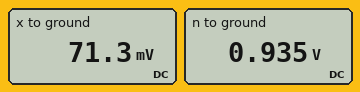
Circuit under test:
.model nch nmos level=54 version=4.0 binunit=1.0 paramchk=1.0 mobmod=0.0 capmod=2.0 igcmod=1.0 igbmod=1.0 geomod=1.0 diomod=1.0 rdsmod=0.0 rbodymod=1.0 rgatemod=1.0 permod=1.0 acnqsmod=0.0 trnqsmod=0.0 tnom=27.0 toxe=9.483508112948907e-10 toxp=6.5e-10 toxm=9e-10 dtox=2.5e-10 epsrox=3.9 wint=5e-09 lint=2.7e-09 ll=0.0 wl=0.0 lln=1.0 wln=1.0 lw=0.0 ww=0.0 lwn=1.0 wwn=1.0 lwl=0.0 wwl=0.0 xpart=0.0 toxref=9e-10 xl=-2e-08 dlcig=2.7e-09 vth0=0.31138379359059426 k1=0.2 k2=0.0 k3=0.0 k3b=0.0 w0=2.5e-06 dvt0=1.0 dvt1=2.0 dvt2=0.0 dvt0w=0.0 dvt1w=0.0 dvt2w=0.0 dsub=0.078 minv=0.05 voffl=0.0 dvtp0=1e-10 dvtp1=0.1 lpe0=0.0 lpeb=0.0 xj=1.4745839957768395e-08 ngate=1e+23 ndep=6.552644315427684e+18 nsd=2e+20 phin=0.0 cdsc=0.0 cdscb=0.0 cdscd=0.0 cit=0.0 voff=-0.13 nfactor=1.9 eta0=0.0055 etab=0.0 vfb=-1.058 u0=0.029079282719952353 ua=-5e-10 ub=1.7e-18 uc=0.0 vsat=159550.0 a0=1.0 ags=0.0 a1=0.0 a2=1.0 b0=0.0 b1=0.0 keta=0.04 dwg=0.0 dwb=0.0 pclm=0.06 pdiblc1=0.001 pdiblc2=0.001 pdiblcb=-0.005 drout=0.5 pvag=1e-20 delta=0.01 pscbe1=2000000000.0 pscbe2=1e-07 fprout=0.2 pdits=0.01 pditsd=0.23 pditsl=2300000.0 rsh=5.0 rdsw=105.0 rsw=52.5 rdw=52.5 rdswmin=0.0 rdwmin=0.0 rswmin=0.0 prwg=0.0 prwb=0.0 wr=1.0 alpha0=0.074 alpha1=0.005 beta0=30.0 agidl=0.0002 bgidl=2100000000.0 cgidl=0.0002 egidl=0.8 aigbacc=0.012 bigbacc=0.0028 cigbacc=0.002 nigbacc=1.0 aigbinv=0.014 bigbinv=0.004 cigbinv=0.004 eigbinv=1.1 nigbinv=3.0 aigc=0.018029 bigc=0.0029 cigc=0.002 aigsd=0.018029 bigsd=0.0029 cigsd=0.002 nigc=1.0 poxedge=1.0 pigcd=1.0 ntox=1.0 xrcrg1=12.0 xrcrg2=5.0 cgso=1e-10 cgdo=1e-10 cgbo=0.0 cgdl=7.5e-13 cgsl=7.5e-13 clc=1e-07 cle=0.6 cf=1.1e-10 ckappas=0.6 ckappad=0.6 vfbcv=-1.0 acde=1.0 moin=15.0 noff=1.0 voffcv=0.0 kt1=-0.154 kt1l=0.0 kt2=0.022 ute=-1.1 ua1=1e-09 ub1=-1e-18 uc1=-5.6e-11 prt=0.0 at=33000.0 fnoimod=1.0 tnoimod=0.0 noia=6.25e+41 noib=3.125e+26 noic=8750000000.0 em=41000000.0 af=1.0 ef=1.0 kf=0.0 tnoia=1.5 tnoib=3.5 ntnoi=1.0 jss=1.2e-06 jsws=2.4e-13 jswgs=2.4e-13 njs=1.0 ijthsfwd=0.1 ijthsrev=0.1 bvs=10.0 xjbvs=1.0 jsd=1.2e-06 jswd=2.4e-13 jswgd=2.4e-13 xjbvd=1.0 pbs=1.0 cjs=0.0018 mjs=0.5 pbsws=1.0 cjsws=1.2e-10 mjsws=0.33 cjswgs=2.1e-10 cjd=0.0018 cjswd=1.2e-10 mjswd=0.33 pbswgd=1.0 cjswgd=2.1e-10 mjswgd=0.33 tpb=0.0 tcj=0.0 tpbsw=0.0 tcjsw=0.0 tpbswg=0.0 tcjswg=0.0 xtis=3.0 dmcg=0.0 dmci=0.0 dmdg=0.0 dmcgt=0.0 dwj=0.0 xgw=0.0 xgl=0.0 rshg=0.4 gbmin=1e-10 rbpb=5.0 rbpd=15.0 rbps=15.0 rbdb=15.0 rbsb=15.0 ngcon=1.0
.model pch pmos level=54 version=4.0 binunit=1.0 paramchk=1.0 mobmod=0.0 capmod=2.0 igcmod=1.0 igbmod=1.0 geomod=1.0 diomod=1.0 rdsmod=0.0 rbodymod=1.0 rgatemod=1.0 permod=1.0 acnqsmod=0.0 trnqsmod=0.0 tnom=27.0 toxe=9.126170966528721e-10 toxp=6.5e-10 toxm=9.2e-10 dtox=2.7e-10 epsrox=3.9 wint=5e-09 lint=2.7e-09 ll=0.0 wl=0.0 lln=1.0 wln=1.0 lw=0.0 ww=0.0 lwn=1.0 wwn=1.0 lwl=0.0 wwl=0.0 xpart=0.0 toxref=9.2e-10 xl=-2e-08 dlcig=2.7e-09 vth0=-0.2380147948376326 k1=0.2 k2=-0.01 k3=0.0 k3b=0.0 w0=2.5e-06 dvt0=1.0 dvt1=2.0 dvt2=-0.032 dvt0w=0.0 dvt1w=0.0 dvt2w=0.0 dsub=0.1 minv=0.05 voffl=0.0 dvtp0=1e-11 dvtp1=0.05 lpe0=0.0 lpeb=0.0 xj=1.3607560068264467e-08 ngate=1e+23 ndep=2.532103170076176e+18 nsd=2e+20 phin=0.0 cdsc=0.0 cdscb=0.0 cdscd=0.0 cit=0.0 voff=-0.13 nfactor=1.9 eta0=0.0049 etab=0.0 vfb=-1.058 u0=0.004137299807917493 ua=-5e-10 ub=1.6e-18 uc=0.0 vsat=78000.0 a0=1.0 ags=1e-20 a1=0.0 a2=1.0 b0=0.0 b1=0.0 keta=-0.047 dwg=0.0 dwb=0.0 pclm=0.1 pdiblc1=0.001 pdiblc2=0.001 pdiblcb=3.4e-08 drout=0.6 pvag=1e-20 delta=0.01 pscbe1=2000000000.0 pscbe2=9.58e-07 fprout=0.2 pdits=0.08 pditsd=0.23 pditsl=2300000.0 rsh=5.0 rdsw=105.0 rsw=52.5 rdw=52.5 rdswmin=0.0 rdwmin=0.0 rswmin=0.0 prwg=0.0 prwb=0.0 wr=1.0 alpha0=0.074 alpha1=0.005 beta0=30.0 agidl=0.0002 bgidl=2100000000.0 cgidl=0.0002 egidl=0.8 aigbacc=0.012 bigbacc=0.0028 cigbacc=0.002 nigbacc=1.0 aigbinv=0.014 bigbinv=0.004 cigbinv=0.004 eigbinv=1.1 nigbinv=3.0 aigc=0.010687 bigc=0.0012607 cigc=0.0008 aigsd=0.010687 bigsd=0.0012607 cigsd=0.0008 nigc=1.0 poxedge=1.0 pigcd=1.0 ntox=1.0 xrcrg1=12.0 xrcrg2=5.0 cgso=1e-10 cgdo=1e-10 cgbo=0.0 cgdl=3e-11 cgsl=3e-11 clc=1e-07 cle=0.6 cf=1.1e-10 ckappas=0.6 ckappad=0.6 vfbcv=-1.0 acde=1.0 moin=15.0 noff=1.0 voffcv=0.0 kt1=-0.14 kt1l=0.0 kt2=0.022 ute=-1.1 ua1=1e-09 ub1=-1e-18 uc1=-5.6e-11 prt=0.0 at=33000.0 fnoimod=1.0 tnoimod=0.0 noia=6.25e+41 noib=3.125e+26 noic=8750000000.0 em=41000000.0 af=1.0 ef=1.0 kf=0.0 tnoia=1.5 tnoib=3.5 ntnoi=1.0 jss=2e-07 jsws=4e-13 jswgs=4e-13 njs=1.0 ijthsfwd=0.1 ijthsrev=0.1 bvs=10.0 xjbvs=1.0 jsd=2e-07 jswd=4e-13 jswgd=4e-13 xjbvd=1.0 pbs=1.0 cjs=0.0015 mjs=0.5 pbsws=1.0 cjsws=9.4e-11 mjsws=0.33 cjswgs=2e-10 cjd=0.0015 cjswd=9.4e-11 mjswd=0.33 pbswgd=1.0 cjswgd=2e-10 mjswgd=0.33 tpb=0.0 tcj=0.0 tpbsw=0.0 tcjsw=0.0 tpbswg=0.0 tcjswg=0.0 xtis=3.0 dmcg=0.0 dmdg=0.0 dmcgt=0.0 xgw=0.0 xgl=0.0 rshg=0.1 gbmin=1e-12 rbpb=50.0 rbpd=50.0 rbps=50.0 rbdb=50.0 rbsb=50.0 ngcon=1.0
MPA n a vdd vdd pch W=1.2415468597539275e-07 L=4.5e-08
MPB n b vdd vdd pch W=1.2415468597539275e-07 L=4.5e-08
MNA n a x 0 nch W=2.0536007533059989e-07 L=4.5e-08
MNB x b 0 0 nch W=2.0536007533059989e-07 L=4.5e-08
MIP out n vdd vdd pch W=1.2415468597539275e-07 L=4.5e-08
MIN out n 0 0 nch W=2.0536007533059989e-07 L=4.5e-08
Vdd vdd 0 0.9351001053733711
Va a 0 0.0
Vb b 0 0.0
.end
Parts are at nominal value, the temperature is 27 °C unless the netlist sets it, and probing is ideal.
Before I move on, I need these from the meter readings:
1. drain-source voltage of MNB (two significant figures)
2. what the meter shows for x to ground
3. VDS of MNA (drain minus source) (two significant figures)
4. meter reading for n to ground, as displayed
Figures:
71 mV
71.3 mV
860 mV
0.935 V
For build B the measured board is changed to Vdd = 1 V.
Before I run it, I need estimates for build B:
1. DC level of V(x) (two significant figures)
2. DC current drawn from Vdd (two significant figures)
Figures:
76 mV
160 nA
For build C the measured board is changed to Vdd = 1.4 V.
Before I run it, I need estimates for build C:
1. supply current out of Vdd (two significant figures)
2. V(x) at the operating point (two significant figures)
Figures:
1.7 µA
100 mV
